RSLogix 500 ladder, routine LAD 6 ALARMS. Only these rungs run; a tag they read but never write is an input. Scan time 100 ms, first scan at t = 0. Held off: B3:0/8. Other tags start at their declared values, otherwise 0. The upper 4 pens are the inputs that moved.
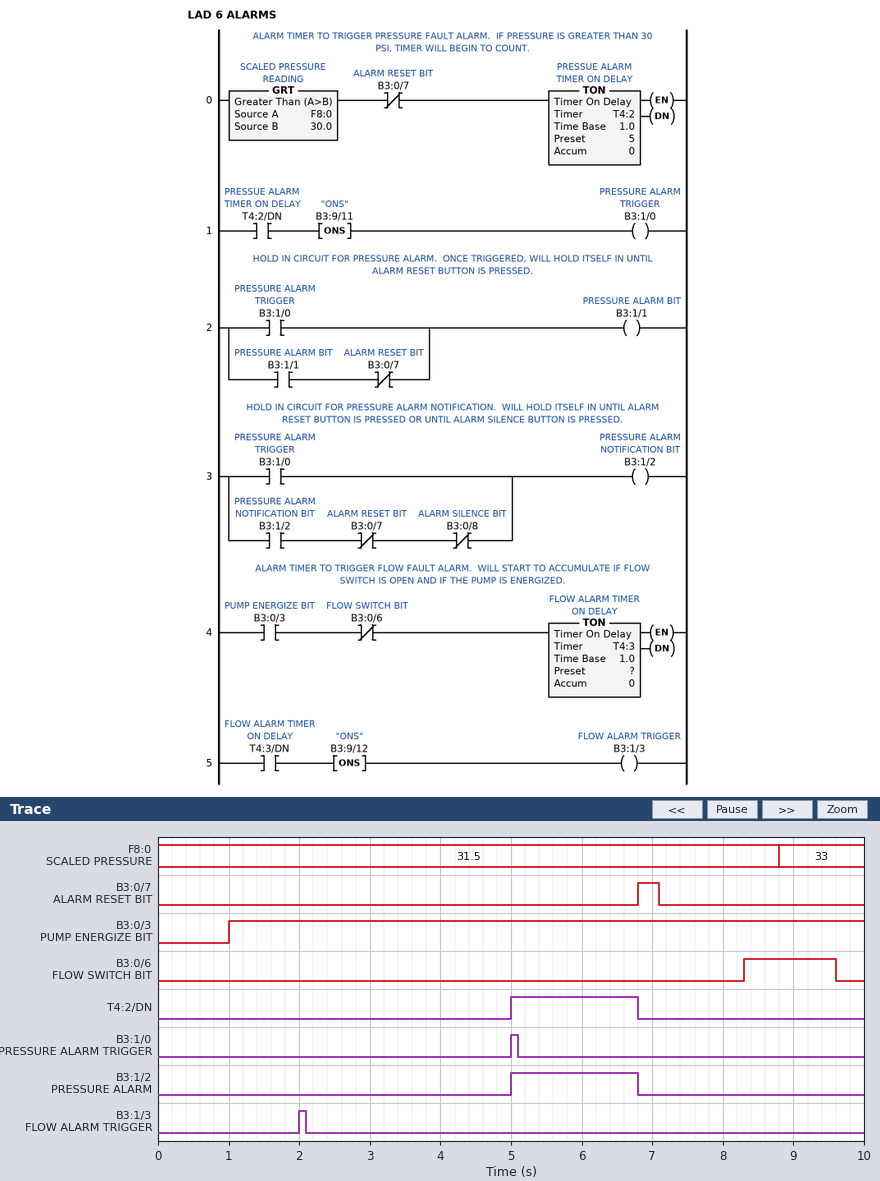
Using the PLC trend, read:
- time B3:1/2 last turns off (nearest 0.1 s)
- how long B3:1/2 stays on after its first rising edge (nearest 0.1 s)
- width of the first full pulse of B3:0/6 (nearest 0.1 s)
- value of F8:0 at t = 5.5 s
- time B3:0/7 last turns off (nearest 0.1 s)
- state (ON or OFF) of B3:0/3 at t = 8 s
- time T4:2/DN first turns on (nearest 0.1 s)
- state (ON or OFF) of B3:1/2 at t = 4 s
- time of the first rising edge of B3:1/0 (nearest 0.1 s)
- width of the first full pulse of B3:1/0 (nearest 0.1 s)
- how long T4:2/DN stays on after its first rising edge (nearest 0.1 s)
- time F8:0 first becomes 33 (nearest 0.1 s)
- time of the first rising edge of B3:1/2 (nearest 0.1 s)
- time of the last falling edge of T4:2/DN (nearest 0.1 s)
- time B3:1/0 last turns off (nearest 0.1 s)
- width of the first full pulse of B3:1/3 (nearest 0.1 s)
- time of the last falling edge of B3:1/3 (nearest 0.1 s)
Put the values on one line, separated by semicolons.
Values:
6.8 s; 1.8 s; 1.3 s; 31.5; 7.1 s; ON; 5.0 s; OFF; 5.0 s; 0.1 s; 1.8 s; 8.8 s; 5.0 s; 6.8 s; 5.1 s; 0.1 s; 2.1 s
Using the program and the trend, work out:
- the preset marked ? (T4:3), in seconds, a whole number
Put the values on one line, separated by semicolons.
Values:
1 s
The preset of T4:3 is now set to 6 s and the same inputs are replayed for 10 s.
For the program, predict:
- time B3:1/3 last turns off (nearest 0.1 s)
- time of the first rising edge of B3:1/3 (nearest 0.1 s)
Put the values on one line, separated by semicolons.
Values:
7.1 s; 7.0 s
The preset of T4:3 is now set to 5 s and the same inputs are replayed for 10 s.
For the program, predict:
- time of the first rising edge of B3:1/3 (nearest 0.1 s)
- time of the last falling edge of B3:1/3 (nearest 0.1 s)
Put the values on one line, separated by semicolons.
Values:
6.0 s; 6.1 s
